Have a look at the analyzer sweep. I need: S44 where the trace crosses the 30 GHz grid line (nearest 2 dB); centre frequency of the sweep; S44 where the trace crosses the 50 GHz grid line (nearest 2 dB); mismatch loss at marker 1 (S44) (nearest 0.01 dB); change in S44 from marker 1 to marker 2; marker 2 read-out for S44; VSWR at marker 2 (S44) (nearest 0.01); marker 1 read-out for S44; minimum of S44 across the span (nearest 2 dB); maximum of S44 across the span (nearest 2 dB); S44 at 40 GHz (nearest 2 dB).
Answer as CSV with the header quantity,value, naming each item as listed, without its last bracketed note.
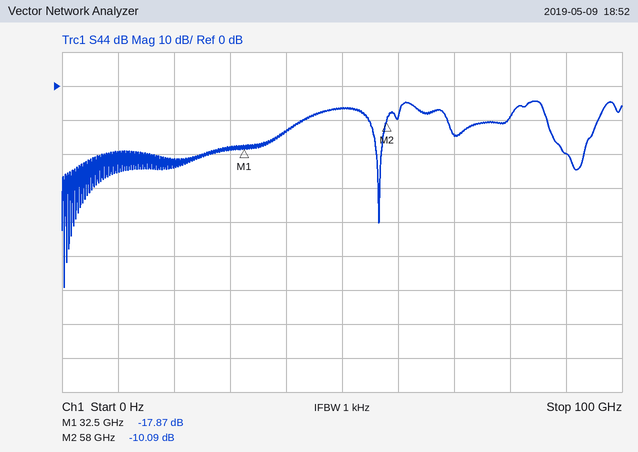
quantity,value
S44 where the trace crosses the 30 GHz grid line,-18 dB
centre frequency of the sweep,50 GHz
S44 where the trace crosses the 50 GHz grid line,-6 dB
mismatch loss at marker 1 (S44),0.07 dB
change in S44 from marker 1 to marker 2,7.78 dB
marker 2 read-out for S44,-10.09 dB
VSWR at marker 2 (S44),1.91
marker 1 read-out for S44,-17.87 dB
minimum of S44 across the span,-60 dB
maximum of S44 across the span,-4 dB
S44 at 40 GHz,-14 dB
